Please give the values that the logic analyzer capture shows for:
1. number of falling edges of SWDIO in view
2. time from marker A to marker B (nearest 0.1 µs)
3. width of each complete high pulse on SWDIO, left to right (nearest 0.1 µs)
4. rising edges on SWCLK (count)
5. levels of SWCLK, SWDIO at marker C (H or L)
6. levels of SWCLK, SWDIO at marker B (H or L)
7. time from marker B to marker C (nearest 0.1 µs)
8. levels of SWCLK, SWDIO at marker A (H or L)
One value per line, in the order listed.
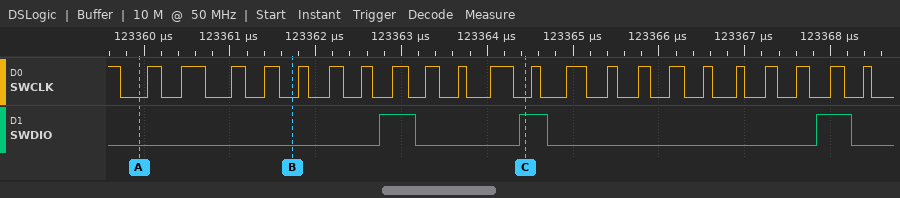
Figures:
3
1.8 µs
0.4 µs, 0.3 µs, 0.4 µs
22
SWCLK=L, SWDIO=H
SWCLK=L, SWDIO=L
2.7 µs
SWCLK=L, SWDIO=L
